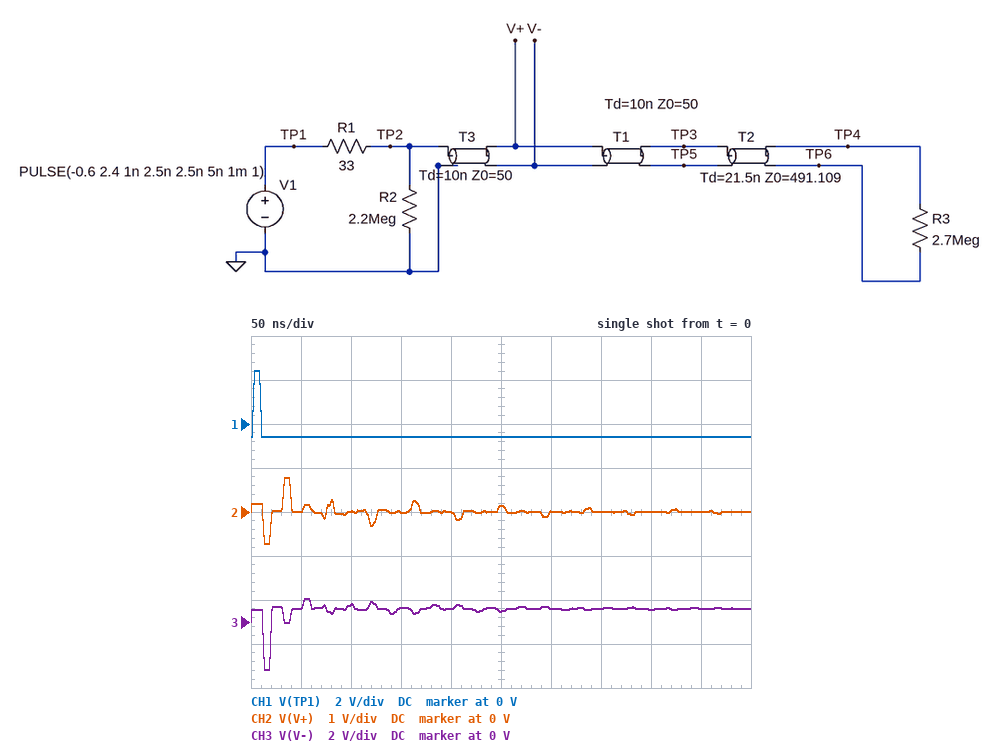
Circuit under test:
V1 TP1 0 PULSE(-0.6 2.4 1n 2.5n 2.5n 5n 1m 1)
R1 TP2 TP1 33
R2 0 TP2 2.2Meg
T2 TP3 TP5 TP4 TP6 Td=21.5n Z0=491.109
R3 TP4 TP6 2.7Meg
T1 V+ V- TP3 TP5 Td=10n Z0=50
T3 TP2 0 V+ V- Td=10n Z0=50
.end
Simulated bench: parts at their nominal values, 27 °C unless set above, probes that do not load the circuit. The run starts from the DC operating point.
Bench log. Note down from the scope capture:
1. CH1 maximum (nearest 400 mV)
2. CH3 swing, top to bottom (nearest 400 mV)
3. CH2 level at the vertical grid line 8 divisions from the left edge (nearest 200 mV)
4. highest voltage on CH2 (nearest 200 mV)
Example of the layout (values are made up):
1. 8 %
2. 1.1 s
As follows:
1. 2.4 V
2. 3.2 V
3. 0 V
4. 800 mV
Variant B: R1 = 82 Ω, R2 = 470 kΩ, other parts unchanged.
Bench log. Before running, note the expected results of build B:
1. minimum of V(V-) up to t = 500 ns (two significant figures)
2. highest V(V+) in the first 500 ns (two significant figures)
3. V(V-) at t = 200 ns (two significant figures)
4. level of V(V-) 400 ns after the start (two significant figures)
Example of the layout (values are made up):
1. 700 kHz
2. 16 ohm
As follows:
1. -900 mV
2. 6.1 mV
3. 590 mV
4. 610 mV
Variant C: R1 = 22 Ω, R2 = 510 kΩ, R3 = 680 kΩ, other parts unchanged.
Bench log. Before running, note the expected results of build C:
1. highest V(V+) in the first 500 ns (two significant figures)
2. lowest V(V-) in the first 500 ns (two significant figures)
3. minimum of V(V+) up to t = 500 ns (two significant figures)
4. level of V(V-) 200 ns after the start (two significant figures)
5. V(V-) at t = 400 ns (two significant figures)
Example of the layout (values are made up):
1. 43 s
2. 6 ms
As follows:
1. 890 mV
2. -2.5 V
3. -830 mV
4. 610 mV
5. 530 mV
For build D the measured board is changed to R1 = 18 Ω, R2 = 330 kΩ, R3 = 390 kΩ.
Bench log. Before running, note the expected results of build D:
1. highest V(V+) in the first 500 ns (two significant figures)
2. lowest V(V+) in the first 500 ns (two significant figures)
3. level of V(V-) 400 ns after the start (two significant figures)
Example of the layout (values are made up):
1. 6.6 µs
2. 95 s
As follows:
1. 940 mV
2. -880 mV
3. 520 mV
